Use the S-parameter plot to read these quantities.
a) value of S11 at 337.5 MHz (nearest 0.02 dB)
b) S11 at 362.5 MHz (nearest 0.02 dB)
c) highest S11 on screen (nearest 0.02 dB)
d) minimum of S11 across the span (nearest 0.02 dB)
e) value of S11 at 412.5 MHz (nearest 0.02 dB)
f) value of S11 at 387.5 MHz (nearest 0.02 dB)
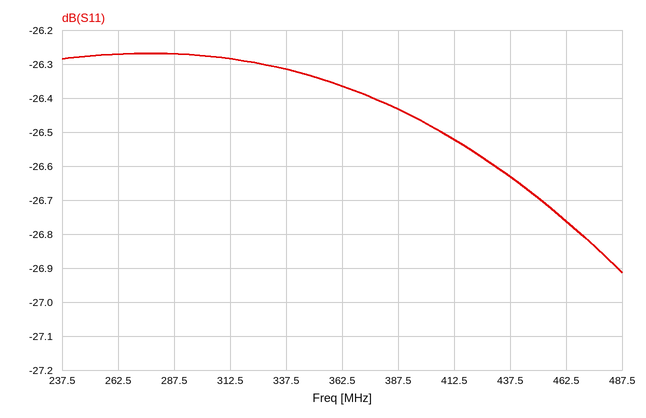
-26.32 dB
-26.36 dB
-26.26 dB
-26.92 dB
-26.52 dB
-26.44 dB
